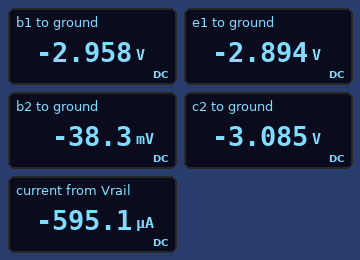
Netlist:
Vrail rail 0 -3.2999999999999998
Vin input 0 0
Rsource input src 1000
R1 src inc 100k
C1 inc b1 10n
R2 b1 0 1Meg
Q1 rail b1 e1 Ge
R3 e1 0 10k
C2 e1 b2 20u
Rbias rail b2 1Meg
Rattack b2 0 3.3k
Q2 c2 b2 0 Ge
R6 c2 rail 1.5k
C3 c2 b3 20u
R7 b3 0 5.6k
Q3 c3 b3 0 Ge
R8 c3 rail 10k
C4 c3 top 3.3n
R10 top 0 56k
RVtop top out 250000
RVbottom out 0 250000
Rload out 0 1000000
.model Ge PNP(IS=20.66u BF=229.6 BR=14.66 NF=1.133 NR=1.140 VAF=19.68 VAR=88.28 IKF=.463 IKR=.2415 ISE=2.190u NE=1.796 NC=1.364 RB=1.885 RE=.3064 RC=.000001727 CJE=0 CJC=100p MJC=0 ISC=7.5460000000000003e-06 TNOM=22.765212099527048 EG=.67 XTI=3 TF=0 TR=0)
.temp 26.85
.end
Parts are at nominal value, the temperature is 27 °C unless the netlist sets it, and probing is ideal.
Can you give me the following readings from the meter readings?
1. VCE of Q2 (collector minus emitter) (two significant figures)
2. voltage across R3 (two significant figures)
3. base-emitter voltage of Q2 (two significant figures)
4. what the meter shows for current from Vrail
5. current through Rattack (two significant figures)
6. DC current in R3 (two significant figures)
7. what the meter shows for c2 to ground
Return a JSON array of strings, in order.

["-3.1 V", "2.9 V", "-38 mV", "-595.1 µA", "12 µA", "290 µA", "-3.085 V"]
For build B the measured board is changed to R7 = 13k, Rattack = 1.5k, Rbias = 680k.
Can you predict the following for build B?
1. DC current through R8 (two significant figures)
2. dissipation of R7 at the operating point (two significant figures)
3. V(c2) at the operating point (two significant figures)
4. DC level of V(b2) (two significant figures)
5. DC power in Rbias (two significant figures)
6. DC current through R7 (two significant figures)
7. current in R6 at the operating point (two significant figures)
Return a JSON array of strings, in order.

["250 µA", "260 nW", "-3.2 V", "-23 mV", "16 µW", "4.5 µA", "90 µA"]
